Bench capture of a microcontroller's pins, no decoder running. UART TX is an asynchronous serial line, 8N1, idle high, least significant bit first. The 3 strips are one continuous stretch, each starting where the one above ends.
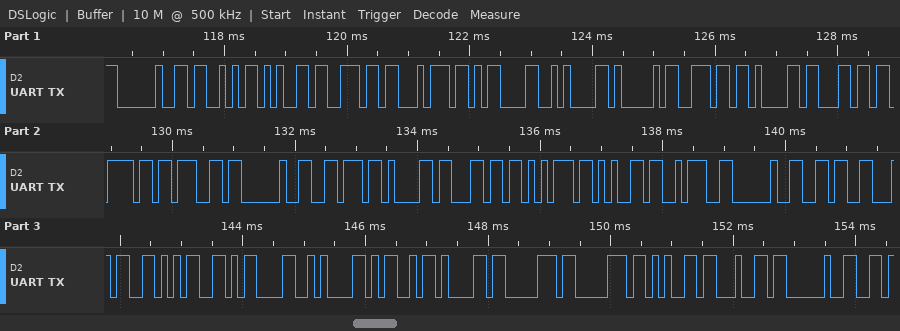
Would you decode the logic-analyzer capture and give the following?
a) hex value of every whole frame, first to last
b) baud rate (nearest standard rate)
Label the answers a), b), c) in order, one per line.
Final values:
a) 0x20 0x53 0x65 0x6E 0x74 0x0D 0x0A 0x41 0x6E 0x61 0x6C 0x6F 0x67 0x20 0x76 0x61 0x6C 0x75 0x65 0x3A 0x20 0x36 0x34 0x35 0x0D 0x0A 0x4D 0x61 0x70 0x70 0x65 0x64 0x20
b) 9600 baud
